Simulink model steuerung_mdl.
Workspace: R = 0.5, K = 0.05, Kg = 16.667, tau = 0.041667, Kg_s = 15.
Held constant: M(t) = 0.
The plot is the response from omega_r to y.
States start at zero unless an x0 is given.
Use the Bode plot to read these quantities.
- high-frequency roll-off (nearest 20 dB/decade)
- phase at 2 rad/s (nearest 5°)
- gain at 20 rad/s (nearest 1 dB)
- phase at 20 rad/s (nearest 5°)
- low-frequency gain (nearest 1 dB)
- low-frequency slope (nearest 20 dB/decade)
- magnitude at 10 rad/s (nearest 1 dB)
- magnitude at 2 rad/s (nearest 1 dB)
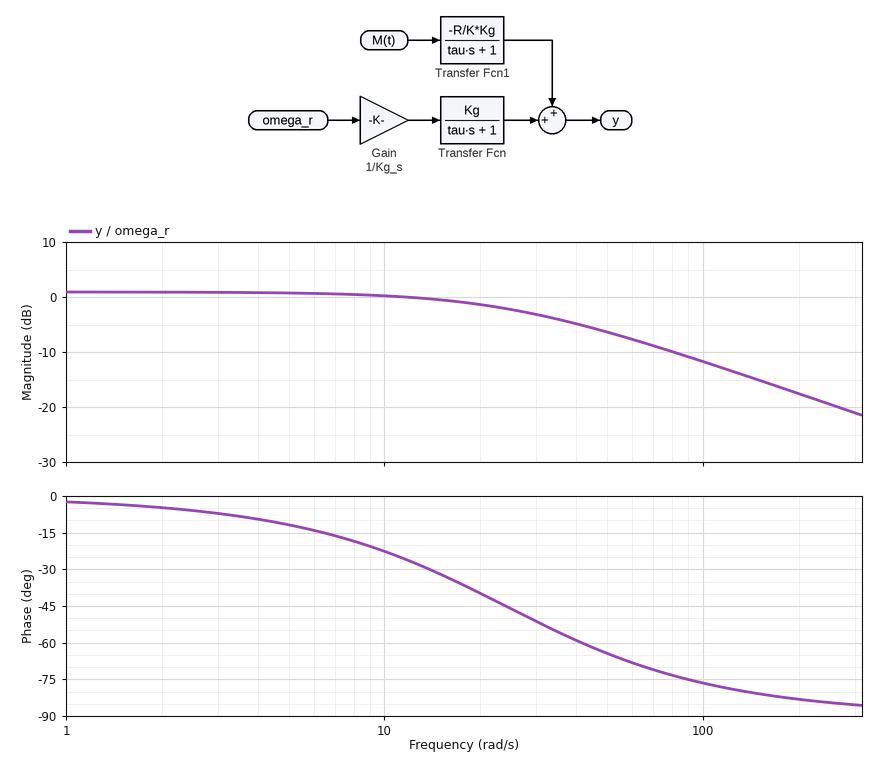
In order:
-20 dB/decade
-5°
-1 dB
-40°
1 dB
0 dB/decade
0 dB
1 dB
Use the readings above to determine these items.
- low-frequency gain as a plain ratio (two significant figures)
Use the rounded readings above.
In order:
1.1
